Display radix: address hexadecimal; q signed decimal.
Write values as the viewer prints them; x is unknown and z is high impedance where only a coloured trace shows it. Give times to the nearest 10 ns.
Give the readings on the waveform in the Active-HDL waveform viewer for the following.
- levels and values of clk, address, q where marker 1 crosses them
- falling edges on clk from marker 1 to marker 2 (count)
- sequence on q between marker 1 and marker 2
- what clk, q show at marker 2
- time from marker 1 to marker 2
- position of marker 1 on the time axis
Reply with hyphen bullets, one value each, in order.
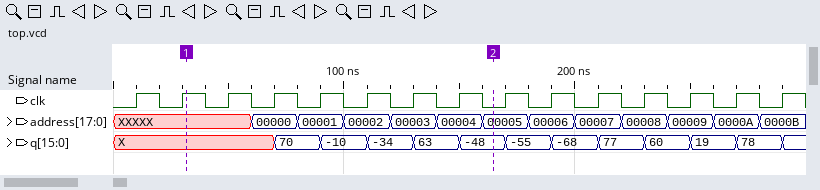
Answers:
- clk=1, address=XXXXX, q=X
- 7
- X, 70, -10, -34, 63, -48
- clk=0, q=-48
- 130 ns
- 30 ns
